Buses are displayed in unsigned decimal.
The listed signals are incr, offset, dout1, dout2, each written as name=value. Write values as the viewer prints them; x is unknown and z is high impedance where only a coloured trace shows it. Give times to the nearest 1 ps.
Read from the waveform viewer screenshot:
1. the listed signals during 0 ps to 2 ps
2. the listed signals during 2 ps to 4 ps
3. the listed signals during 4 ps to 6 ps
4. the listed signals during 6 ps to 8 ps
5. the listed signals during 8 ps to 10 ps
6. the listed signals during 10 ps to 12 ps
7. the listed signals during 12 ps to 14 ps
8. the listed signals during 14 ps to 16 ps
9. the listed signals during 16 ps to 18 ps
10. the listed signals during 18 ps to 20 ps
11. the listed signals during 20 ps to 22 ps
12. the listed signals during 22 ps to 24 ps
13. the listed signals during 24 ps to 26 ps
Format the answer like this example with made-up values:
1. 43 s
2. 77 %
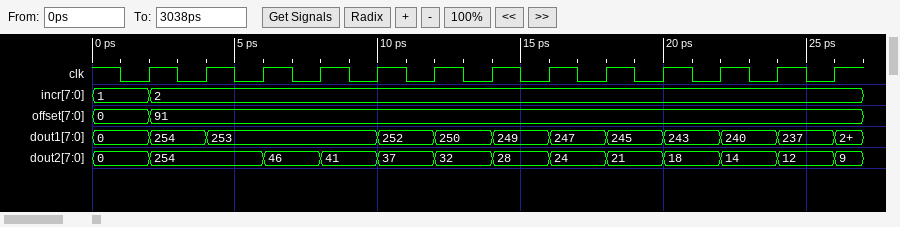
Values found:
1. incr=1, offset=0, dout1=0, dout2=0
2. incr=2, offset=91, dout1=254, dout2=254
3. incr=2, offset=91, dout1=253, dout2=254
4. incr=2, offset=91, dout1=253, dout2=46
5. incr=2, offset=91, dout1=253, dout2=41
6. incr=2, offset=91, dout1=252, dout2=37
7. incr=2, offset=91, dout1=250, dout2=32
8. incr=2, offset=91, dout1=249, dout2=28
9. incr=2, offset=91, dout1=247, dout2=24
10. incr=2, offset=91, dout1=245, dout2=21
11. incr=2, offset=91, dout1=243, dout2=18
12. incr=2, offset=91, dout1=240, dout2=14
13. incr=2, offset=91, dout1=237, dout2=12
